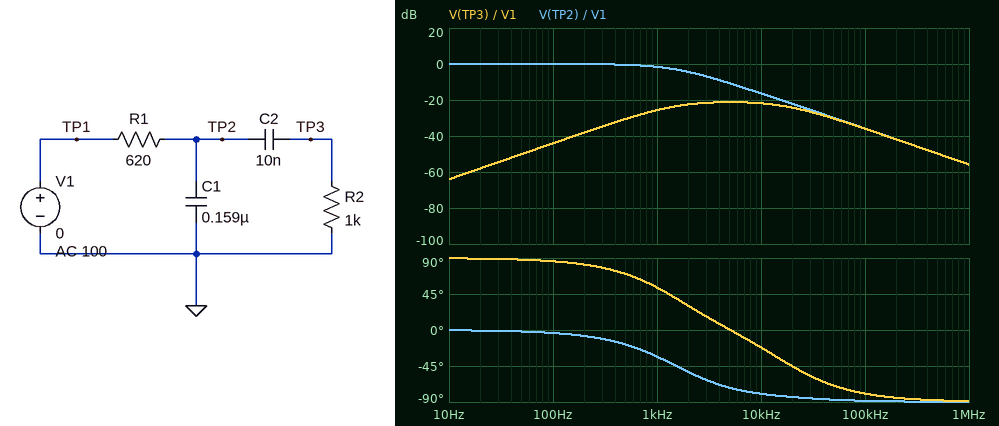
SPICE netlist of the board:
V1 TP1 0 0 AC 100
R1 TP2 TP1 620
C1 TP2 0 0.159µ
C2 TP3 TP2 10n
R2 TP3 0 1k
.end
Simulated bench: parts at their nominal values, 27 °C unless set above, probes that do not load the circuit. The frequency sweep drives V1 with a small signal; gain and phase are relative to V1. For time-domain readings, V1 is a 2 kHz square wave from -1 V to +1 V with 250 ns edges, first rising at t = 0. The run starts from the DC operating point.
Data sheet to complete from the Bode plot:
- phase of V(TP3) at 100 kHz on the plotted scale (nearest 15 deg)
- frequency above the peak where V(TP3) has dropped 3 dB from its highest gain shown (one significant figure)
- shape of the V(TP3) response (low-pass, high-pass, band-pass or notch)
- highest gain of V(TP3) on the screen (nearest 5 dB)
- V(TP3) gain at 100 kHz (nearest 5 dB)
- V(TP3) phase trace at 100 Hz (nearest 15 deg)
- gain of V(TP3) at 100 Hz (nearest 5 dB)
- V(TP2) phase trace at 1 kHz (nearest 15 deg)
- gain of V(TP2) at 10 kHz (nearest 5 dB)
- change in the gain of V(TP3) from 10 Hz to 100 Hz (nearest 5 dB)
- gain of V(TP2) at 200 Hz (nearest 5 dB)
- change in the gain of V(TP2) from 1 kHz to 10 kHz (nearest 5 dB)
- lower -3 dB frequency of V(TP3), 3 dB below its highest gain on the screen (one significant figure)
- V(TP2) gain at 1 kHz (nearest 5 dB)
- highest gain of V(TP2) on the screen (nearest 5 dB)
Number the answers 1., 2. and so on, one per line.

1. -75 deg
2. 20 kHz
3. band-pass
4. -20 dB
5. -35 dB
6. 90 deg
7. -45 dB
8. -30 deg
9. -15 dB
10. 20 dB
11. 0 dB
12. -15 dB
13. 1 kHz
14. 0 dB
15. 0 dB
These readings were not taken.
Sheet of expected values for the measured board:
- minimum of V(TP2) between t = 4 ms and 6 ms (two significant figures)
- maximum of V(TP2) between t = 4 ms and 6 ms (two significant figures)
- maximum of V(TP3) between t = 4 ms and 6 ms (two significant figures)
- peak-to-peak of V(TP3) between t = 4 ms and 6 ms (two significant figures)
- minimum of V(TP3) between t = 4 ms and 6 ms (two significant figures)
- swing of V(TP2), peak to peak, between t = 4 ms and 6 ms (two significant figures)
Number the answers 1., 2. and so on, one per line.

1. -830 mV
2. 830 mV
3. 140 mV
4. 270 mV
5. -140 mV
6. 1.7 V
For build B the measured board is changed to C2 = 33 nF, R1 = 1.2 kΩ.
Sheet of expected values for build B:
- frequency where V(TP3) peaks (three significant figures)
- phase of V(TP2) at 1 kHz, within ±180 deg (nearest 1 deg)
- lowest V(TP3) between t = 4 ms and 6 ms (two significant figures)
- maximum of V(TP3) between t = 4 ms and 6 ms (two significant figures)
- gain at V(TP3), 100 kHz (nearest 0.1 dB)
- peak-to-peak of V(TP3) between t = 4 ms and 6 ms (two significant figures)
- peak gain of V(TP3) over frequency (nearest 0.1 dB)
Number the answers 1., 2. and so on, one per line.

1. 2.01 kHz
2. -54 deg
3. -150 mV
4. 150 mV
5. -41.6 dB
6. 300 mV
7. -18.0 dB
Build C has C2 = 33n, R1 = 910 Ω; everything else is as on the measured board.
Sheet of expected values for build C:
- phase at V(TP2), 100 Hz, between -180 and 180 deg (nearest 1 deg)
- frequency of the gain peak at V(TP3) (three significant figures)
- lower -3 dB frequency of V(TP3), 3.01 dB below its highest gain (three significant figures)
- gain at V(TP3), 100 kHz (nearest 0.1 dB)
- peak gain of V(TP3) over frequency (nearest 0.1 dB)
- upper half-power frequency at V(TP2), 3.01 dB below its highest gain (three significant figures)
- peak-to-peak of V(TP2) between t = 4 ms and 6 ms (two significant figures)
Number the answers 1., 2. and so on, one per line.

1. -6 deg
2. 2.30 kHz
3. 696 Hz
4. -39.2 dB
5. -16.0 dB
6. 888 Hz
7. 1.2 V
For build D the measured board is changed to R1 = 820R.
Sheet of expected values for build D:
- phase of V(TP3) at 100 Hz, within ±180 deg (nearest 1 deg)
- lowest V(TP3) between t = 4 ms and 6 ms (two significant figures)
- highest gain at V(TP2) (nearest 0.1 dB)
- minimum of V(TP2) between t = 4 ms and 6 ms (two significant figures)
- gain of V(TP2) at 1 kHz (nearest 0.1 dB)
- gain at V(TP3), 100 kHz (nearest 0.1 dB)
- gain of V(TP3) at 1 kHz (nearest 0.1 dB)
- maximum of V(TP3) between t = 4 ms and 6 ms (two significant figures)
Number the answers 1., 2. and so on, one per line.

1. 85 deg
2. -100 mV
3. 0 dB
4. -720 mV
5. -2.5 dB
6. -38.4 dB
7. -26.5 dB
8. 100 mV
